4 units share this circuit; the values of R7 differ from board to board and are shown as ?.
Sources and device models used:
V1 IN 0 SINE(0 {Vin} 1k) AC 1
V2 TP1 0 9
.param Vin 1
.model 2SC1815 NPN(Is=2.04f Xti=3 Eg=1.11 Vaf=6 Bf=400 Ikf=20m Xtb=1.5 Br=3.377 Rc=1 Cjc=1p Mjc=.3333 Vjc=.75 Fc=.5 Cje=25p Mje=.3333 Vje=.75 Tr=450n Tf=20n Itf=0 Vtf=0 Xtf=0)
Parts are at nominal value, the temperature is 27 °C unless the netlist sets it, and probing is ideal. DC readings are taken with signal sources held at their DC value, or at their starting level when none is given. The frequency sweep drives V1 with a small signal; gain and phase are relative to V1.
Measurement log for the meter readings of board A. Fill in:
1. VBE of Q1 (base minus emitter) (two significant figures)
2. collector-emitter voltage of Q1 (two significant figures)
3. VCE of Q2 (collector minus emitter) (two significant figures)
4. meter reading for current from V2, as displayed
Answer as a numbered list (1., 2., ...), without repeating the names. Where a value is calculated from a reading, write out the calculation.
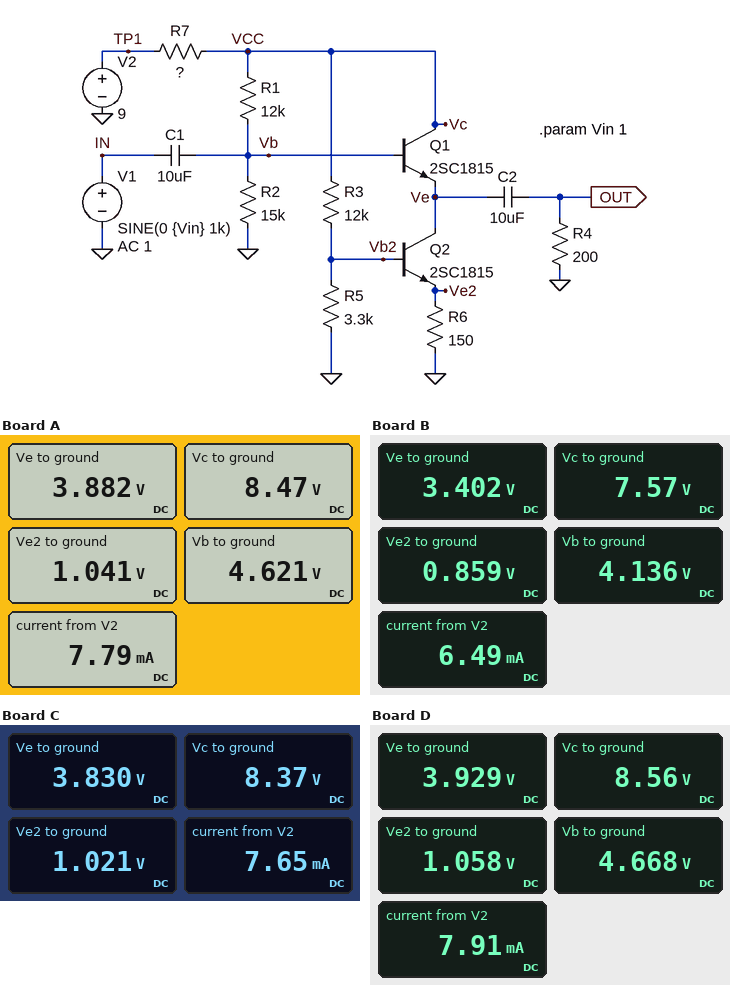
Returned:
1. 4.621 V - 3.882 V = 740 mV
2. 8.47 V - 3.882 V = 4.6 V
3. 3.882 V - 1.041 V = 2.8 V
4. 7.79 mA
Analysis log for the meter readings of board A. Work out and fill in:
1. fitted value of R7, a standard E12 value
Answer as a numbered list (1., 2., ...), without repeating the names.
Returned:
1. 68 Ω
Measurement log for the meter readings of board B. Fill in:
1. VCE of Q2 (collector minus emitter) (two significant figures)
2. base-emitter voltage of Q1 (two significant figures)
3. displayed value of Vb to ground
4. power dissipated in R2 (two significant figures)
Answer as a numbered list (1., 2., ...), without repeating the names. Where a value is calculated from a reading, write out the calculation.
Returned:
1. 3.402 V - 859 mV = 2.5 V
2. 4.136 V - 3.402 V = 730 mV
3. 4.136 V
4. (4.136 V)^2 / 15 kΩ = 1.1 mW
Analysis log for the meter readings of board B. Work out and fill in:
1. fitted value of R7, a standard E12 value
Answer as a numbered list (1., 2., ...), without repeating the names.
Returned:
1. 220 Ω
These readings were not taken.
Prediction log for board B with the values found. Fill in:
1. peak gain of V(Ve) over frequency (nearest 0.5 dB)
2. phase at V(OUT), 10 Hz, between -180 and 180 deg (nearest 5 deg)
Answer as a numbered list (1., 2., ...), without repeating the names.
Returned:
1. 0 dB
2. 95 deg
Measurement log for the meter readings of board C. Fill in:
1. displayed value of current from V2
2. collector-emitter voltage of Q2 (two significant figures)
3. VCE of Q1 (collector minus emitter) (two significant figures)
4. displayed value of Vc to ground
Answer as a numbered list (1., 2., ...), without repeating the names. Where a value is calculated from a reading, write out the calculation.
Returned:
1. 7.65 mA
2. 3.83 V - 1.021 V = 2.8 V
3. 8.37 V - 3.83 V = 4.5 V
4. 8.37 V
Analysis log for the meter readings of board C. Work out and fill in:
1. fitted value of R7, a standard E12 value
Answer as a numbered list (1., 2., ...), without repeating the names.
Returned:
1. 82 Ω
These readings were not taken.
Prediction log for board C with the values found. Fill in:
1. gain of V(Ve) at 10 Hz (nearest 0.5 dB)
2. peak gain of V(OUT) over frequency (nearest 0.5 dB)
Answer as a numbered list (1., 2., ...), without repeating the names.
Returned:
1. -0.5 dB
2. 0 dB
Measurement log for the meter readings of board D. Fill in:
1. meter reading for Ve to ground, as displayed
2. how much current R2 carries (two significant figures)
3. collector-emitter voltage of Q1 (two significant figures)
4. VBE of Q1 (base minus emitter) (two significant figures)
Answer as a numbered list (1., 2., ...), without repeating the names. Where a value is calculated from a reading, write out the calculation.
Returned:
1. 3.929 V
2. (4.668 V) / 15 kΩ = 310 µA
3. 8.56 V - 3.929 V = 4.6 V
4. 4.668 V - 3.929 V = 740 mV
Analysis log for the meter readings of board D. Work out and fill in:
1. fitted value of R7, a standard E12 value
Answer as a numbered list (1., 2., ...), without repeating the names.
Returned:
1. 56 Ω
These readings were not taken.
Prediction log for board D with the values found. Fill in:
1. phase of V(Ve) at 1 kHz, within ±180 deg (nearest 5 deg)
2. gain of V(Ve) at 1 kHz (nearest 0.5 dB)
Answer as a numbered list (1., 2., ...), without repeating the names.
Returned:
1. 0 deg
2. 0 dB
